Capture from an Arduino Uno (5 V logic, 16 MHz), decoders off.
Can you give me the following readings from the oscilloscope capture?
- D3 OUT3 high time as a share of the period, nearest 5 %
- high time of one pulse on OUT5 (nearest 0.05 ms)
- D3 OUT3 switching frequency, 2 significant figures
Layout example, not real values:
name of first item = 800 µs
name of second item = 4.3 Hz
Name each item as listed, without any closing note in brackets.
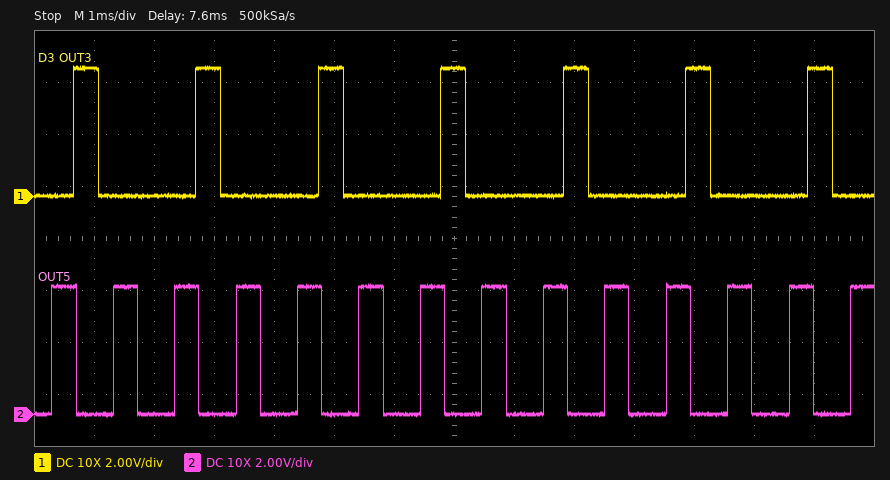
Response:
D3 OUT3 high time as a share of the period, nearest 5 % = 20 %
high time of one pulse on OUT5 = 0.40 ms
D3 OUT3 switching frequency, 2 significant figures = 490 Hz
